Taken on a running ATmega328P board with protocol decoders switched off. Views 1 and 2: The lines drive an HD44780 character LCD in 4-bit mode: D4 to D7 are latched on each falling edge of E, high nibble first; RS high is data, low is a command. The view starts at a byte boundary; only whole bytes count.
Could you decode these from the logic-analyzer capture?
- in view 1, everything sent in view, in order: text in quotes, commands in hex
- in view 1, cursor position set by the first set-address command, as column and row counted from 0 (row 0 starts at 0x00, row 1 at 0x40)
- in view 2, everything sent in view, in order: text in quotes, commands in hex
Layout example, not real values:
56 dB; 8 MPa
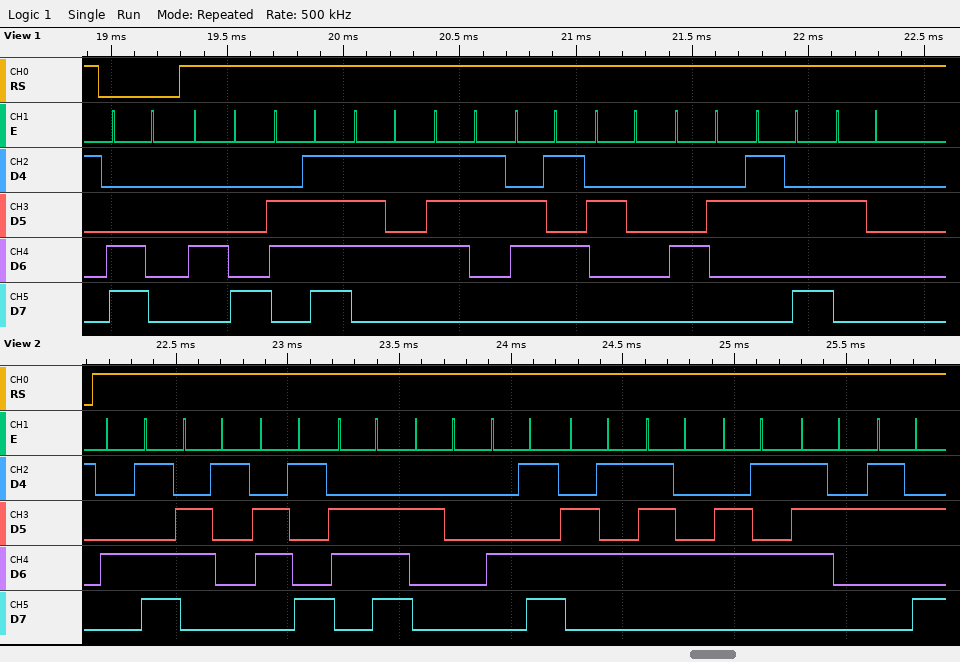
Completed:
0xC0 "House B: "; column 0, row 1; "Main Meter:"
